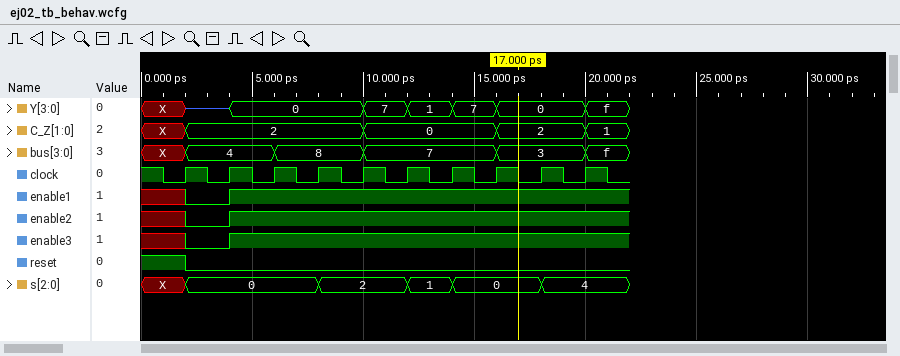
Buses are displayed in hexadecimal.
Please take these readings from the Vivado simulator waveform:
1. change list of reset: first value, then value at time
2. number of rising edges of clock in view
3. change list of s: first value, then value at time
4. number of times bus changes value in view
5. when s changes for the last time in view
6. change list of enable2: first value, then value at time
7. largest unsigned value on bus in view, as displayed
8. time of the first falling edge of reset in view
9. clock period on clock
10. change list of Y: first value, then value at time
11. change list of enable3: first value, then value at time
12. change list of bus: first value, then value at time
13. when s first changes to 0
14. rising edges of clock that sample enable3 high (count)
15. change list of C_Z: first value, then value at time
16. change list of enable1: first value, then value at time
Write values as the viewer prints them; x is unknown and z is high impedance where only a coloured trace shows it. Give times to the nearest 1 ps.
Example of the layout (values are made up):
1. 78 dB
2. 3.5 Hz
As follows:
1. 1, 0 at 2 ps
2. 10
3. X, 0 at 2 ps, 2 at 8 ps, 1 at 12 ps, 0 at 14 ps, 4 at 18 ps
4. 5
5. 18 ps
6. x, 0 at 2 ps, 1 at 4 ps
7. f
8. 2 ps
9. 2 ps
10. X, z at 2 ps, 0 at 4 ps, 7 at 10 ps, 1 at 12 ps, 7 at 14 ps, 0 at 16 ps, f at 20 ps
11. x, 0 at 2 ps, 1 at 4 ps
12. X, 4 at 2 ps, 8 at 6 ps, 7 at 10 ps, 3 at 16 ps, f at 20 ps
13. 2 ps
14. 8
15. X, 2 at 2 ps, 0 at 10 ps, 2 at 16 ps, 1 at 20 ps
16. x, 0 at 2 ps, 1 at 4 ps
